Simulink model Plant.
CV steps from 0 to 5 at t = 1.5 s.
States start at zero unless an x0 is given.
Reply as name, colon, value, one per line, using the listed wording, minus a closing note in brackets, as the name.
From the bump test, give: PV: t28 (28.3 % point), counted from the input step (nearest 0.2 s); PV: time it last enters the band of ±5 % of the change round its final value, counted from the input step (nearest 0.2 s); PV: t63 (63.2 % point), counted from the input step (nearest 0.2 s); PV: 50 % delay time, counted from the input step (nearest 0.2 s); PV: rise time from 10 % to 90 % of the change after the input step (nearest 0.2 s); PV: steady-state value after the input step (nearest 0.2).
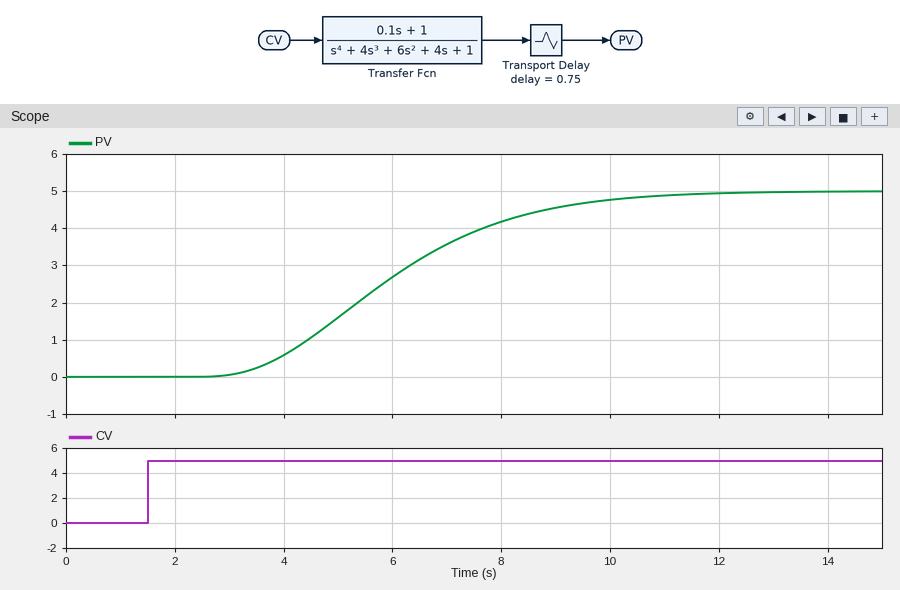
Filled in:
PV: t28 (28.3 % point), counted from the input step: 3.4 s
PV: time it last enters the band of ±5 % of the change round its final value, counted from the input step: 8.4 s
PV: t63 (63.2 % point), counted from the input step: 5.0 s
PV: 50 % delay time, counted from the input step: 4.4 s
PV: rise time from 10 % to 90 % of the change after the input step: 5.0 s
PV: steady-state value after the input step: 5.0
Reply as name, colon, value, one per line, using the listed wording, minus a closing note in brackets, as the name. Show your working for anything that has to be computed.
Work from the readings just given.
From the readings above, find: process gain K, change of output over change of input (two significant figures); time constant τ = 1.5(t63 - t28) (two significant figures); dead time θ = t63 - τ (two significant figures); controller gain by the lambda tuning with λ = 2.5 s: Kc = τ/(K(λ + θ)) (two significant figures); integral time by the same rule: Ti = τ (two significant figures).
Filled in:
process gain K, change of output over change of input: (5 - 0) / 5 = 1.0
time constant τ = 1.5(t63 - t28): 1.5 × (5 - 3.4) = 2.4 s
dead time θ = t63 - τ: 5 - 2.4 = 2.6 s
controller gain by the lambda tuning with λ = 2.5 s: Kc = τ/(K(λ + θ)): 2.4 / (1 × (2.5 + 2.6)) = 0.47
integral time by the same rule: Ti = τ: 2.4 s
